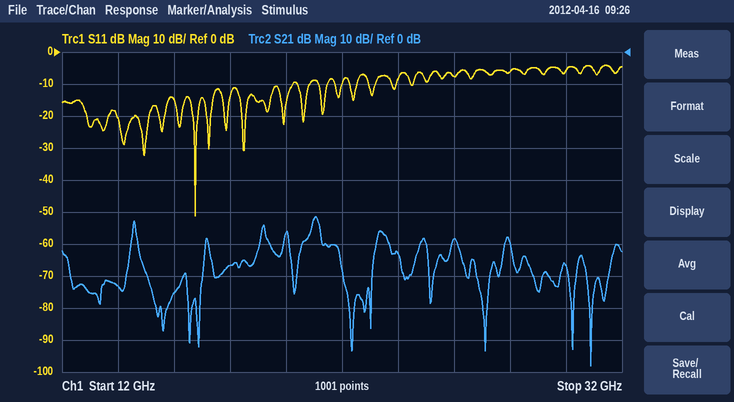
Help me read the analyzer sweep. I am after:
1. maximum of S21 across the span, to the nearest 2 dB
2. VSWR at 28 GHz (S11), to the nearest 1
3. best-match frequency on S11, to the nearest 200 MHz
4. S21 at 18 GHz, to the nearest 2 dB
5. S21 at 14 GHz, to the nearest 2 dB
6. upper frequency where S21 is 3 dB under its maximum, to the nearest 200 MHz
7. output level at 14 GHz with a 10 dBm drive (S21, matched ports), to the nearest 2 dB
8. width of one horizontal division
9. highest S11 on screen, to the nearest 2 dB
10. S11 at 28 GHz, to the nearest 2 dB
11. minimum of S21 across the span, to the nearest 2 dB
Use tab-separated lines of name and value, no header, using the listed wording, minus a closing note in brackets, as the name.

maximum of S21 across the span, to the nearest 2 dB	-52 dB
VSWR at 28 GHz (S11), to the nearest 1	3
best-match frequency on S11, to the nearest 200 MHz	16.8 GHz
S21 at 18 GHz, to the nearest 2 dB	-66 dB
S21 at 14 GHz, to the nearest 2 dB	-74 dB
upper frequency where S21 is 3 dB under its maximum, to the nearest 200 MHz	21.2 GHz
output level at 14 GHz with a 10 dBm drive (S21, matched ports), to the nearest 2 dB	-64 dBm
width of one horizontal division	2 GHz
highest S11 on screen, to the nearest 2 dB	-4 dB
S11 at 28 GHz, to the nearest 2 dB	-6 dB
minimum of S21 across the span, to the nearest 2 dB	-98 dB
